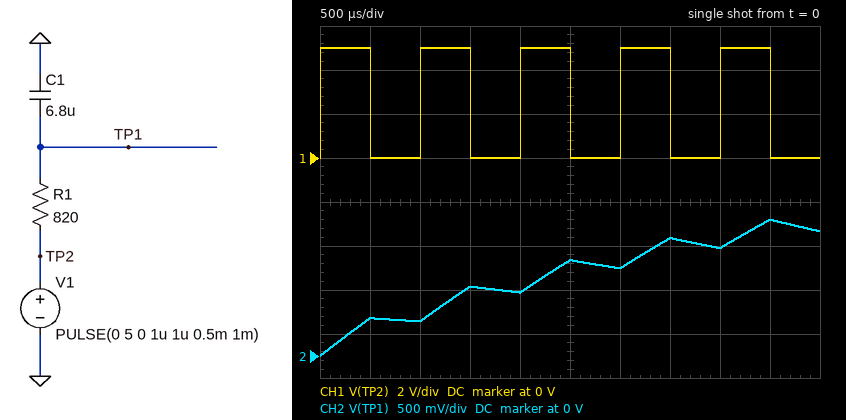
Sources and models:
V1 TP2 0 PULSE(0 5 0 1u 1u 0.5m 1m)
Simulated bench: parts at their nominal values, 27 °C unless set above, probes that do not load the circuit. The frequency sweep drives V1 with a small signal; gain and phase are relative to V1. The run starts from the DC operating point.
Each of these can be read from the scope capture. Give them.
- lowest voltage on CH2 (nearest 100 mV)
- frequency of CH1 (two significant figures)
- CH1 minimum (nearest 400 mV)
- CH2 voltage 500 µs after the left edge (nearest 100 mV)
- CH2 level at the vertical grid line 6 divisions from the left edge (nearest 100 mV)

0 V
1.0 kHz
0 V
400 mV
1.0 V
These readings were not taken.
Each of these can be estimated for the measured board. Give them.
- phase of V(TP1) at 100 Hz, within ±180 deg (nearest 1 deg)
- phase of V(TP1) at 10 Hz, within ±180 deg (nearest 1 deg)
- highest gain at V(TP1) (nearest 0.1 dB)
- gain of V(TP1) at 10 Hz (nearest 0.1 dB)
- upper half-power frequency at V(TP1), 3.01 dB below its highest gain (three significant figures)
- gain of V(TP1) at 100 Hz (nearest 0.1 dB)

-74 deg
-19 deg
0 dB
-0.5 dB
28.5 Hz
-11.2 dB
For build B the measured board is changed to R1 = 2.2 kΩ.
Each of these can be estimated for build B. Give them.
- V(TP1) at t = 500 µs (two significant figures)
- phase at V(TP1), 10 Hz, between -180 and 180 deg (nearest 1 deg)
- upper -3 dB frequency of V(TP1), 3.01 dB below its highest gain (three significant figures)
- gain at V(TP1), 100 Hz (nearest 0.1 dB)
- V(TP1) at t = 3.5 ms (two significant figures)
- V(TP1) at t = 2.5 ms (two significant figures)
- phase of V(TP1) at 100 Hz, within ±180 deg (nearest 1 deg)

160 mV
-43 deg
10.6 Hz
-19.5 dB
600 mV
460 mV
-84 deg
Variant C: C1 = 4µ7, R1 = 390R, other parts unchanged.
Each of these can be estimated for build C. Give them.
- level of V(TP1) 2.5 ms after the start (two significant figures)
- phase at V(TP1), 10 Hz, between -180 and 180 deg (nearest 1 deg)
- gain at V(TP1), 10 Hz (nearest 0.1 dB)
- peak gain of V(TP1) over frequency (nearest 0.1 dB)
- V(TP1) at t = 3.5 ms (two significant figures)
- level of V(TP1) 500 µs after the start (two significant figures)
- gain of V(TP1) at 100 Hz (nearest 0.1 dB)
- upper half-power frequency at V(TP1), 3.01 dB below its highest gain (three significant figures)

2.3 V
-7 deg
-0.1 dB
0 dB
2.5 V
1.2 V
-3.7 dB
86.8 Hz
